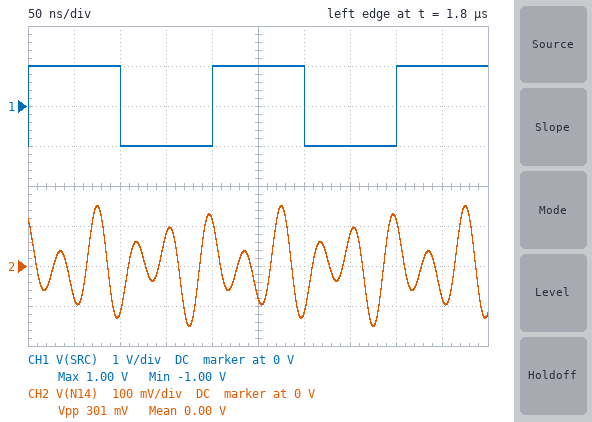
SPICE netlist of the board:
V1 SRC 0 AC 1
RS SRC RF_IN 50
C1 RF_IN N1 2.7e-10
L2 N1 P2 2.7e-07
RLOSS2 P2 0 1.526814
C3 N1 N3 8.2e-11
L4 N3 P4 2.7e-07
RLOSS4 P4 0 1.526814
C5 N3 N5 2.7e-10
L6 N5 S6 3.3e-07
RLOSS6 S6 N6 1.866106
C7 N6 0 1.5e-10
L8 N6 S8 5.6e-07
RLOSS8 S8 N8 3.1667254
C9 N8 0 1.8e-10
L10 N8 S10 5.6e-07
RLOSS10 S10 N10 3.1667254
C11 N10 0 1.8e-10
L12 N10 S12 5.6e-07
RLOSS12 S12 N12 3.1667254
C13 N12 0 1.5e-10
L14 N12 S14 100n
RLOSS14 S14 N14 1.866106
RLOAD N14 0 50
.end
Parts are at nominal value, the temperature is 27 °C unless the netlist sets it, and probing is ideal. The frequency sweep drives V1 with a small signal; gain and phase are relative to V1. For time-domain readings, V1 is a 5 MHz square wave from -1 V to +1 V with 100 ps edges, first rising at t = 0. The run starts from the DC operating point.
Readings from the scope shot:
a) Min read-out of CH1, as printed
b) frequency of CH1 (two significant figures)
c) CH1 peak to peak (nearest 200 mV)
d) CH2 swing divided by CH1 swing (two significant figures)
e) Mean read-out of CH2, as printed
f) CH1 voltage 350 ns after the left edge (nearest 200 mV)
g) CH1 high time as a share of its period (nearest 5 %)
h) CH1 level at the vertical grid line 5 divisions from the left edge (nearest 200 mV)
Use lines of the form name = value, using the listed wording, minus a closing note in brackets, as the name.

Min read-out of CH1, as printed = -1.00 V
frequency of CH1 = 5.0 MHz
CH1 peak to peak = 2.0 V
CH2 swing divided by CH1 swing = 0.15
Mean read-out of CH2, as printed = 0.00 V
CH1 voltage 350 ns after the left edge = -1.0 V
CH1 high time as a share of its period = 50 %
CH1 level at the vertical grid line 5 divisions from the left edge = 1.0 V
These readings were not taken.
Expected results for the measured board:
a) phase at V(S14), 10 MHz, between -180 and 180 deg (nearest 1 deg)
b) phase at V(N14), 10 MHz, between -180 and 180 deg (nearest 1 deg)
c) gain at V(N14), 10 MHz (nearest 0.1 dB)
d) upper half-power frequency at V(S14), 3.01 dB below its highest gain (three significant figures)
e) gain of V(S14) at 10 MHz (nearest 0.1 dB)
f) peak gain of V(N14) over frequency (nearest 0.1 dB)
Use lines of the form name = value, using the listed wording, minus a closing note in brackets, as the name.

phase at V(S14), 10 MHz, between -180 and 180 deg = -167 deg
phase at V(N14), 10 MHz, between -180 and 180 deg = -167 deg
gain at V(N14), 10 MHz = -34.8 dB
upper half-power frequency at V(S14), 3.01 dB below its highest gain = 30.3 MHz
gain of V(S14) at 10 MHz = -34.5 dB
peak gain of V(N14) over frequency = -8.5 dB
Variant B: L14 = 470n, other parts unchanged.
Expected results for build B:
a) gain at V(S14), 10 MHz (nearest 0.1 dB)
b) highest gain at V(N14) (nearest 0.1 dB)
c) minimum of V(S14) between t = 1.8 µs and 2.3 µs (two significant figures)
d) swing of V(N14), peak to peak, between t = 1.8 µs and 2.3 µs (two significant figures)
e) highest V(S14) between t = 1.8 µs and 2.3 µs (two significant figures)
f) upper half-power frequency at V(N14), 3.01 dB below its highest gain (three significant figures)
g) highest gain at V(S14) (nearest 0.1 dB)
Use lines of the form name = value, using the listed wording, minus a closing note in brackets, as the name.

gain at V(S14), 10 MHz = -33.7 dB
highest gain at V(N14) = -8.4 dB
minimum of V(S14) between t = 1.8 µs and 2.3 µs = -140 mV
swing of V(N14), peak to peak, between t = 1.8 µs and 2.3 µs = 280 mV
highest V(S14) between t = 1.8 µs and 2.3 µs = 140 mV
upper half-power frequency at V(N14), 3.01 dB below its highest gain = 30.8 MHz
highest gain at V(S14) = -8.1 dB
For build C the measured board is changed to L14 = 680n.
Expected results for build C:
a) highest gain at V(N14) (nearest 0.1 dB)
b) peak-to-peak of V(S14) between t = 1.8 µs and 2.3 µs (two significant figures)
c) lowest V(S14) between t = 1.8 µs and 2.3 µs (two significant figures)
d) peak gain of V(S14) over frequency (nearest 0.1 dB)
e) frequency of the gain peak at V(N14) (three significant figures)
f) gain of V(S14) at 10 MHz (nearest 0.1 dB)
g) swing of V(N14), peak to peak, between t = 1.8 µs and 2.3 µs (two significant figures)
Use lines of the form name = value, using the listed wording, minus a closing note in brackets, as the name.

highest gain at V(N14) = -9.1 dB
peak-to-peak of V(S14) between t = 1.8 µs and 2.3 µs = 260 mV
lowest V(S14) between t = 1.8 µs and 2.3 µs = -130 mV
peak gain of V(S14) over frequency = -8.7 dB
frequency of the gain peak at V(N14) = 25.9 MHz
gain of V(S14) at 10 MHz = -33.3 dB
swing of V(N14), peak to peak, between t = 1.8 µs and 2.3 µs = 250 mV
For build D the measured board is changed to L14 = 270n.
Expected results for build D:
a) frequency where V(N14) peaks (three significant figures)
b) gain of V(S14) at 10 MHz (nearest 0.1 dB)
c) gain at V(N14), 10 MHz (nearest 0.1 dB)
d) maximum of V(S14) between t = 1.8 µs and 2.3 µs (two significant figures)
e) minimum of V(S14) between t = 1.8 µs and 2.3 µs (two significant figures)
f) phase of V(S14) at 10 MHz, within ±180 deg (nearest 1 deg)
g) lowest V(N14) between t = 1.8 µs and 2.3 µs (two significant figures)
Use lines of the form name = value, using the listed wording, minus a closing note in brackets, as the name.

frequency where V(N14) peaks = 26.1 MHz
gain of V(S14) at 10 MHz = -34.1 dB
gain at V(N14), 10 MHz = -34.4 dB
maximum of V(S14) between t = 1.8 µs and 2.3 µs = 150 mV
minimum of V(S14) between t = 1.8 µs and 2.3 µs = -150 mV
phase of V(S14) at 10 MHz, within ±180 deg = -169 deg
lowest V(N14) between t = 1.8 µs and 2.3 µs = -150 mV
